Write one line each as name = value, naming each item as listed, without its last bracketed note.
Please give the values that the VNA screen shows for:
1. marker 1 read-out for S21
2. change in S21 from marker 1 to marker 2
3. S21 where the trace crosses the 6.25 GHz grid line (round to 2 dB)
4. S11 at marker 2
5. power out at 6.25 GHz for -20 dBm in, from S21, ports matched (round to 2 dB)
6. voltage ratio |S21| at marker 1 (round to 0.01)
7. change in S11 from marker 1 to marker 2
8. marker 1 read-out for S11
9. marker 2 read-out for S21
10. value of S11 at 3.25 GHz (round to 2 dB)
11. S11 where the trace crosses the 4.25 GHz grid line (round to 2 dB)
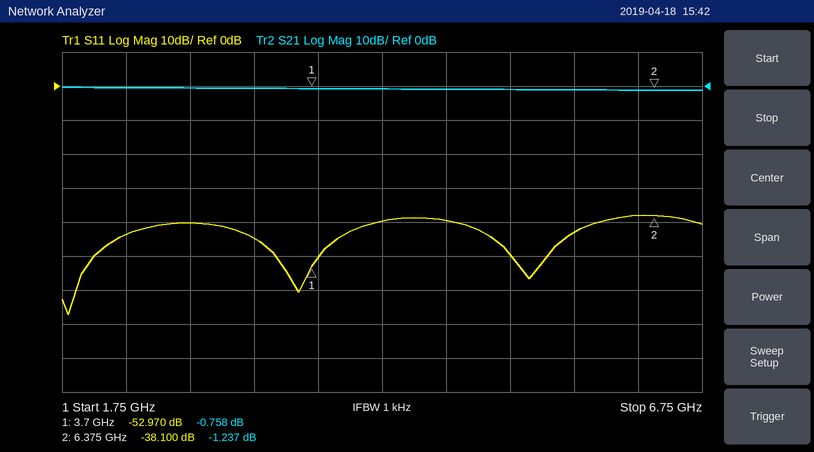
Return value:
marker 1 read-out for S21 = -0.758 dB
change in S21 from marker 1 to marker 2 = -0.479 dB
S21 where the trace crosses the 6.25 GHz grid line = -2 dB
S11 at marker 2 = -38.100 dB
power out at 6.25 GHz for -20 dBm in, from S21, ports matched = -22 dBm
voltage ratio |S21| at marker 1 = 0.92
change in S11 from marker 1 to marker 2 = 14.870 dB
marker 1 read-out for S11 = -52.970 dB
marker 2 read-out for S21 = -1.237 dB
value of S11 at 3.25 GHz = -44 dB
S11 where the trace crosses the 4.25 GHz grid line = -40 dB
